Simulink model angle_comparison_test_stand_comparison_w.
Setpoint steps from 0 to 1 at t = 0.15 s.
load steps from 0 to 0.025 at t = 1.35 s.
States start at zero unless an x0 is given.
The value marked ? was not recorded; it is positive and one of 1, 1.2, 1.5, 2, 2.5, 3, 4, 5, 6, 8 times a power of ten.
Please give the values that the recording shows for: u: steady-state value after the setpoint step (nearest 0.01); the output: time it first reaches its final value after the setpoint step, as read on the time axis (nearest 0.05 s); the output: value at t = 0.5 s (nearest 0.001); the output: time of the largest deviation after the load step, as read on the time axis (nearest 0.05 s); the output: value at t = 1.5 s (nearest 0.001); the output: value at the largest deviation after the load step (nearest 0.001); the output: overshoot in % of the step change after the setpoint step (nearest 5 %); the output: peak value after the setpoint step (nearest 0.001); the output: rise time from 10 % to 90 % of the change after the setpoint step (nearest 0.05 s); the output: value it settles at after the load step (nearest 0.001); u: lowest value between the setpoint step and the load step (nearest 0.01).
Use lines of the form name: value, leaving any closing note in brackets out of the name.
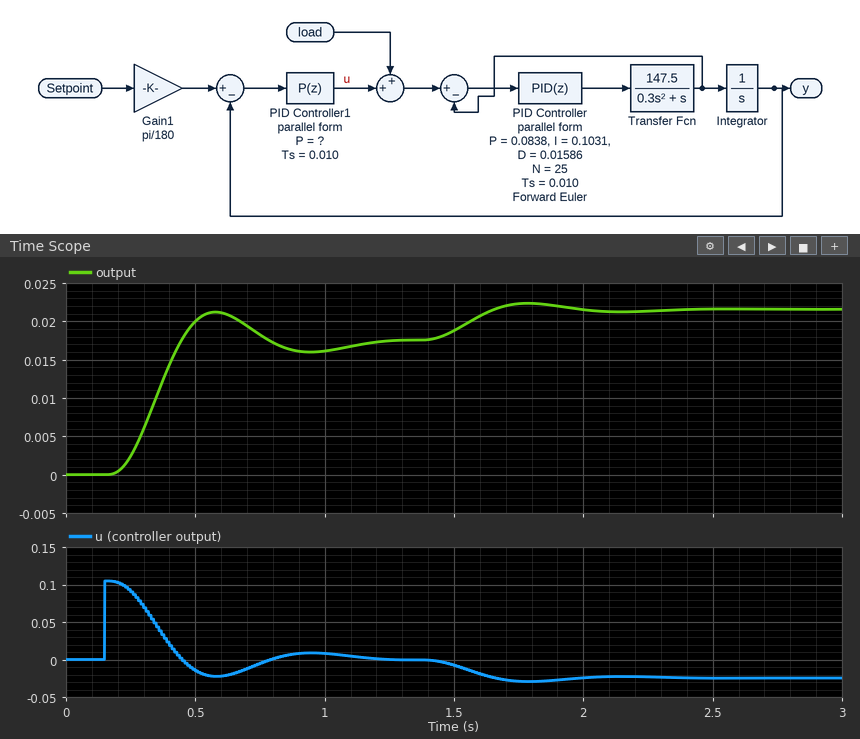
u: steady-state value after the setpoint step: 0.00
the output: time it first reaches its final value after the setpoint step, as read on the time axis: 0.45 s
the output: value at t = 0.5 s: 0.020
the output: time of the largest deviation after the load step, as read on the time axis: 1.80 s
the output: value at t = 1.5 s: 0.019
the output: value at the largest deviation after the load step: 0.022
the output: overshoot in % of the step change after the setpoint step: 20 %
the output: peak value after the setpoint step: 0.021
the output: rise time from 10 % to 90 % of the change after the setpoint step: 0.20 s
the output: value it settles at after the load step: 0.022
u: lowest value between the setpoint step and the load step: -0.02
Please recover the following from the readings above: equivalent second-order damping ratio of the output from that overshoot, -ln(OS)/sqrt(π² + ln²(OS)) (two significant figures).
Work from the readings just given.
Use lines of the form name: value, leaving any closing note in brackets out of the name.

equivalent second-order damping ratio of the output from that overshoot, -ln(OS)/sqrt(π² + ln²(OS)): 0.46
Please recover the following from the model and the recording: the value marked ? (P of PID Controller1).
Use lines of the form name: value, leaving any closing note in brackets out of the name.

the value marked ?: 6
